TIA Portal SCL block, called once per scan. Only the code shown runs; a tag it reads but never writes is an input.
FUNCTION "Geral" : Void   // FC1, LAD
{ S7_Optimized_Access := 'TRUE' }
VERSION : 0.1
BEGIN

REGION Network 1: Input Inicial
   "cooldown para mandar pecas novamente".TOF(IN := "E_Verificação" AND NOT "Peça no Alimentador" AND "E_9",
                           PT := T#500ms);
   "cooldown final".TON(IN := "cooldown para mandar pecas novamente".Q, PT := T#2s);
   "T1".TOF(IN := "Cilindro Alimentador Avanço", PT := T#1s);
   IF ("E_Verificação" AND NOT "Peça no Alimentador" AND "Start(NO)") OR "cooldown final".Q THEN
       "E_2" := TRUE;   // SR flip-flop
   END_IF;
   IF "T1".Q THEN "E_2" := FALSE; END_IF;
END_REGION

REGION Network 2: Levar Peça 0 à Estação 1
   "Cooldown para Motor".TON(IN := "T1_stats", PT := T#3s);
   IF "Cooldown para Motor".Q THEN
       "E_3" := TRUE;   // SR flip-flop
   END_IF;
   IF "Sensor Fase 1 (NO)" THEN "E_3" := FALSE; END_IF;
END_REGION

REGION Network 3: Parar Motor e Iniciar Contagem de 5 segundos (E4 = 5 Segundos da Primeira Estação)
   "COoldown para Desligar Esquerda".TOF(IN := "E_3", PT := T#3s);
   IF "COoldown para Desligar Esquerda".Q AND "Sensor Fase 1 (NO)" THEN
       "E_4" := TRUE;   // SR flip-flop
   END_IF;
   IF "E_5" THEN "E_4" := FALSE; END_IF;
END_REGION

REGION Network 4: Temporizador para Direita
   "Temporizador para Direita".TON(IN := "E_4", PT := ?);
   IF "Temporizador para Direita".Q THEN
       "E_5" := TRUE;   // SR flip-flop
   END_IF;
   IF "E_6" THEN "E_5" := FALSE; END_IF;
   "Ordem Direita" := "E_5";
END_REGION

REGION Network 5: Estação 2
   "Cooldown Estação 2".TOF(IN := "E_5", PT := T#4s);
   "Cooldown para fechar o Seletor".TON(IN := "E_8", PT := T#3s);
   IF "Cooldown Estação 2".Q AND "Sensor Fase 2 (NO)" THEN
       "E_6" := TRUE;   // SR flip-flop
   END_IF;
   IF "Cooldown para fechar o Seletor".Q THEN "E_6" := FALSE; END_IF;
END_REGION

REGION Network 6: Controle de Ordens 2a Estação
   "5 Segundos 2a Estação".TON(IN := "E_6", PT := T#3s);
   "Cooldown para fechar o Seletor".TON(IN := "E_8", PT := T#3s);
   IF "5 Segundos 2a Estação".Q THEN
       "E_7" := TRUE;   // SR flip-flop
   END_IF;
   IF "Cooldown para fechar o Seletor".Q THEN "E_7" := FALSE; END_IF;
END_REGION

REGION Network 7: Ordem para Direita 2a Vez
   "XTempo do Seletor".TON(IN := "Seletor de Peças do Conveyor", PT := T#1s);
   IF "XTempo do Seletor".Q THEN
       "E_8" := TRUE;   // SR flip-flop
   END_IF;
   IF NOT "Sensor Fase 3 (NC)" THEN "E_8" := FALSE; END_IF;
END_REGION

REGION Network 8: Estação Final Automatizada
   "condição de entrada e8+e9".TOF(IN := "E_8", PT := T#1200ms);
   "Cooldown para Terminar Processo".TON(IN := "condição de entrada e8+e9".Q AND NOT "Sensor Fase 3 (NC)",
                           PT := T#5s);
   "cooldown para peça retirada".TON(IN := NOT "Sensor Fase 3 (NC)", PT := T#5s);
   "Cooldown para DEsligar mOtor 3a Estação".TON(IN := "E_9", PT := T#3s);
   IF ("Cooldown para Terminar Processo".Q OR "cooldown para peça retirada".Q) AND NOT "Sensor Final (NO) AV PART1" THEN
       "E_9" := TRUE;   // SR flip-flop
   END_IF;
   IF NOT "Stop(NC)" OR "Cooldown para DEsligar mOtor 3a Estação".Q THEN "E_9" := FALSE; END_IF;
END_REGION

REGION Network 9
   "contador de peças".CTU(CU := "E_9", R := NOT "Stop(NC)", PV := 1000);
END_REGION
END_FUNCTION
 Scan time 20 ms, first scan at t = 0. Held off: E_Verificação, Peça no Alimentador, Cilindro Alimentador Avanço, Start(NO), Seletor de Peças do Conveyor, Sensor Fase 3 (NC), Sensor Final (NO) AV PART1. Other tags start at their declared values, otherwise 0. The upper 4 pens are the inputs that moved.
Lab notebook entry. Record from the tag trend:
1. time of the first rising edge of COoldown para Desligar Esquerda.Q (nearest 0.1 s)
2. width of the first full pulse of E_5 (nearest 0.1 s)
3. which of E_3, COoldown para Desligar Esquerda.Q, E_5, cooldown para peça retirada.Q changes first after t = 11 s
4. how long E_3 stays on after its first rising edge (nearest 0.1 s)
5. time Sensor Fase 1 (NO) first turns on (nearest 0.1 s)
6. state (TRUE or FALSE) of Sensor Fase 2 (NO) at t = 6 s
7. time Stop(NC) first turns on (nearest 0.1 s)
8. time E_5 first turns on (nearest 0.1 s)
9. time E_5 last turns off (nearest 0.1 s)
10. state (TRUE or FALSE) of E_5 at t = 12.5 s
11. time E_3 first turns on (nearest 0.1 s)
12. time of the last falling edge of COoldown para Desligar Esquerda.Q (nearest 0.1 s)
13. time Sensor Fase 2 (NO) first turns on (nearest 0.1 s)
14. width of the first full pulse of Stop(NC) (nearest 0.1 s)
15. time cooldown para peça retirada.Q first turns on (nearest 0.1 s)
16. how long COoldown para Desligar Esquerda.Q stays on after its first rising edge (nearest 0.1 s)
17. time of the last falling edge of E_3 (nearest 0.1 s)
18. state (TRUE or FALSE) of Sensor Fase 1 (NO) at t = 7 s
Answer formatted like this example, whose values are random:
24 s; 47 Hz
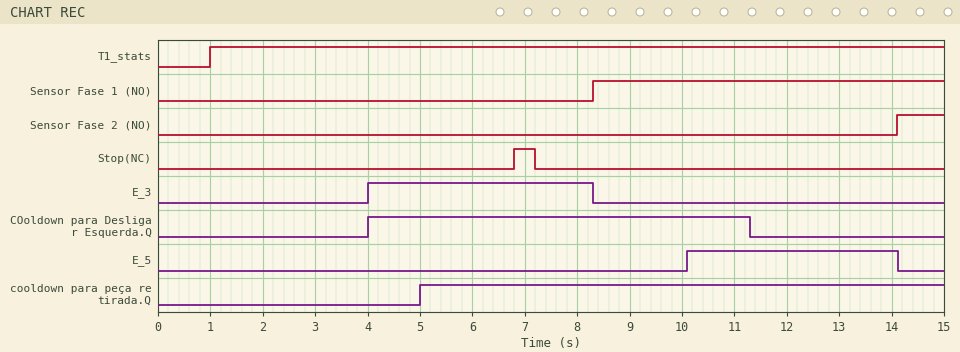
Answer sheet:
4.0 s; 4.0 s; COoldown para Desligar Esquerda.Q; 4.3 s; 8.3 s; FALSE; 6.8 s; 10.1 s; 14.1 s; TRUE; 4.0 s; 11.3 s; 14.1 s; 0.4 s; 5.0 s; 7.3 s; 8.3 s; FALSE
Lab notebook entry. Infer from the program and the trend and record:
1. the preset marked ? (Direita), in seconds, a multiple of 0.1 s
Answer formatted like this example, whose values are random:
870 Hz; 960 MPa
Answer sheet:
1.8 s
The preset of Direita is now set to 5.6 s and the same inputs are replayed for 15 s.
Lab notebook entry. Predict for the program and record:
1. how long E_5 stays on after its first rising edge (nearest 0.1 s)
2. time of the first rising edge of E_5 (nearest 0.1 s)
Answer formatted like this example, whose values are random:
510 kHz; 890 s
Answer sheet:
0.2 s; 13.9 s
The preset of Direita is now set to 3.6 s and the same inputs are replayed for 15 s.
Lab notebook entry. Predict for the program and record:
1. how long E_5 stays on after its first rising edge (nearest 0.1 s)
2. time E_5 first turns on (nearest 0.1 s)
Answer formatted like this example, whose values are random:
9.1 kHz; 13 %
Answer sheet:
2.2 s; 11.9 s
